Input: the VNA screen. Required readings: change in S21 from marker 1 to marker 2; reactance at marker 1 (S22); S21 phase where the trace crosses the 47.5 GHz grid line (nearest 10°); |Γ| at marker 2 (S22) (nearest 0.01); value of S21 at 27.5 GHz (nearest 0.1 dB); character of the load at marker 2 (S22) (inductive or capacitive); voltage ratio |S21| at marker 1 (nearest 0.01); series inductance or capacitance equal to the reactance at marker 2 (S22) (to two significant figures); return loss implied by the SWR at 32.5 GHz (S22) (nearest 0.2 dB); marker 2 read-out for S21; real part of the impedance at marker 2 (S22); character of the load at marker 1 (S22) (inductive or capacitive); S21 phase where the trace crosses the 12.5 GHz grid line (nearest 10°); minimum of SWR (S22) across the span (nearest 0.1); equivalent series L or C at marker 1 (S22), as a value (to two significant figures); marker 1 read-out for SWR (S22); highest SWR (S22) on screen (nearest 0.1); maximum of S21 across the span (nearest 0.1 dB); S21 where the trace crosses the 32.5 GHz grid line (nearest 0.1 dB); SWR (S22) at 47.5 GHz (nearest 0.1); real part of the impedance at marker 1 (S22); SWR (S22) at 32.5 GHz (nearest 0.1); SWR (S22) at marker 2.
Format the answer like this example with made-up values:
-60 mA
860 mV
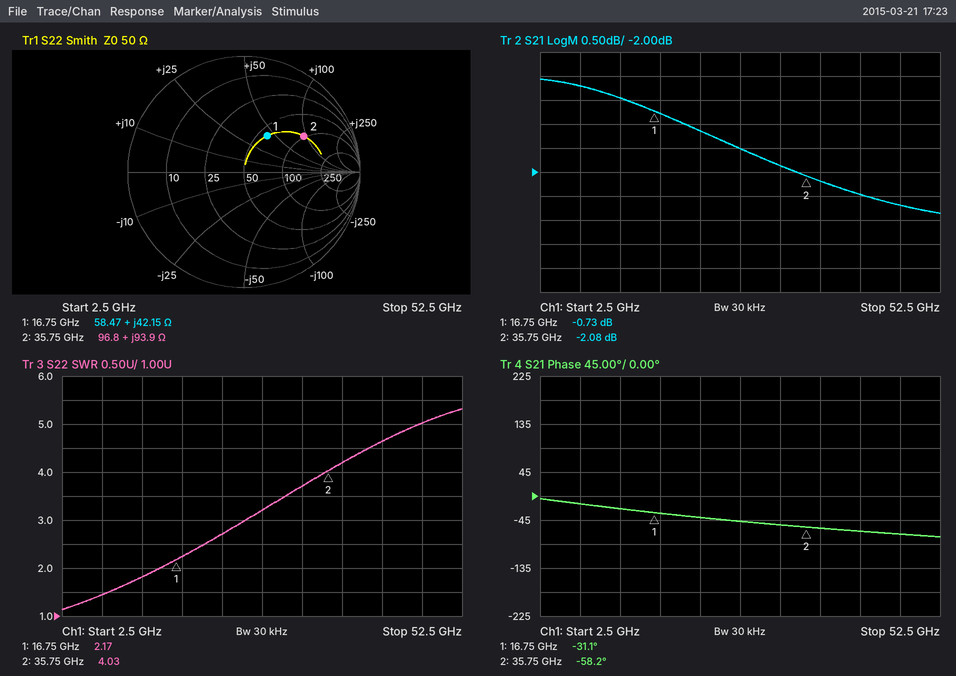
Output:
-1.35 dB
+42.15 Ω
-70°
0.60
-1.5 dB
inductive
0.92
420 pH
4.8 dB
-2.08 dB
96.8 Ω
inductive
-20°
1.1
400 pH
2.17
5.3
-0.1 dB
-1.9 dB
5.0
58.47 Ω
3.7
4.03
